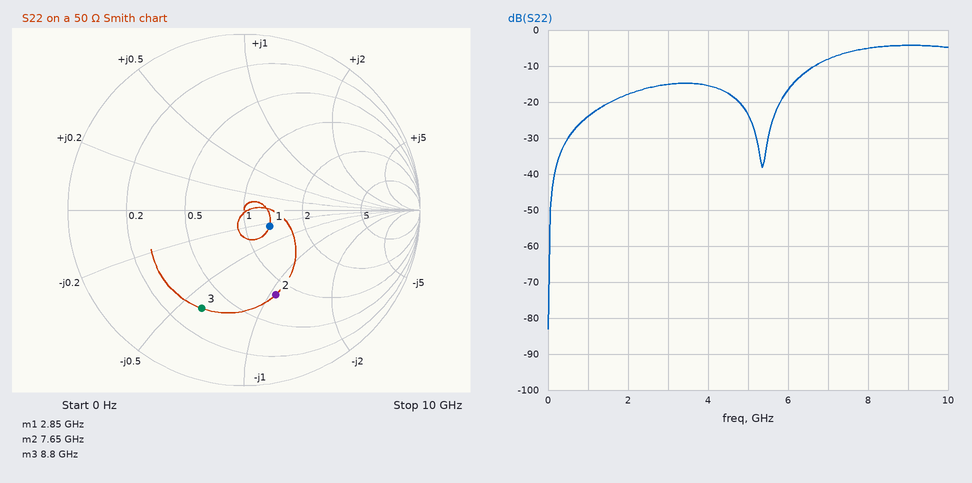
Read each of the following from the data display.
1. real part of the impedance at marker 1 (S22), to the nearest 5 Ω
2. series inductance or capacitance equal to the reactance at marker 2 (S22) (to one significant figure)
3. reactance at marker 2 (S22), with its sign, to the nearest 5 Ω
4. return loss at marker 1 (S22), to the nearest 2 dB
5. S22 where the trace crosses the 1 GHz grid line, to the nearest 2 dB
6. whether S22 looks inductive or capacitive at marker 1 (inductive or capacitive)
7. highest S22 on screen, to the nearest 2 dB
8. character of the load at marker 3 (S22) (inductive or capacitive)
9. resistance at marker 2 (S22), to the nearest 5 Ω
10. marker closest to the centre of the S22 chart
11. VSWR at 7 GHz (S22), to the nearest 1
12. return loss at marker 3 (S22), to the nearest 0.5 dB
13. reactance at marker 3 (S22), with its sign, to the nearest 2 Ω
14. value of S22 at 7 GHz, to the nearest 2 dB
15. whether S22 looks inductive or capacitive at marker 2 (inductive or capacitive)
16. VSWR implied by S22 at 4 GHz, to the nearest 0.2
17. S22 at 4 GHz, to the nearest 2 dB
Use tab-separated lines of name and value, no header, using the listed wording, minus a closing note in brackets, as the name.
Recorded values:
real part of the impedance at marker 1 (S22), to the nearest 5 Ω	65 Ω
series inductance or capacitance equal to the reactance at marker 2 (S22)	400 fF
reactance at marker 2 (S22), with its sign, to the nearest 5 Ω	-55 Ω
return loss at marker 1 (S22), to the nearest 2 dB	16 dB
S22 where the trace crosses the 1 GHz grid line, to the nearest 2 dB	-24 dB
whether S22 looks inductive or capacitive at marker 1	capacitive
highest S22 on screen, to the nearest 2 dB	-4 dB
character of the load at marker 3 (S22)	capacitive
resistance at marker 2 (S22), to the nearest 5 Ω	40 Ω
marker closest to the centre of the S22 chart	marker 1
VSWR at 7 GHz (S22), to the nearest 1	2
return loss at marker 3 (S22), to the nearest 0.5 dB	4.5 dB
reactance at marker 3 (S22), with its sign, to the nearest 2 Ω	-30 Ω
value of S22 at 7 GHz, to the nearest 2 dB	-8 dB
whether S22 looks inductive or capacitive at marker 2	capacitive
VSWR implied by S22 at 4 GHz, to the nearest 0.2	1.4
S22 at 4 GHz, to the nearest 2 dB	-16 dB
